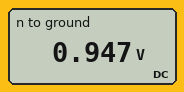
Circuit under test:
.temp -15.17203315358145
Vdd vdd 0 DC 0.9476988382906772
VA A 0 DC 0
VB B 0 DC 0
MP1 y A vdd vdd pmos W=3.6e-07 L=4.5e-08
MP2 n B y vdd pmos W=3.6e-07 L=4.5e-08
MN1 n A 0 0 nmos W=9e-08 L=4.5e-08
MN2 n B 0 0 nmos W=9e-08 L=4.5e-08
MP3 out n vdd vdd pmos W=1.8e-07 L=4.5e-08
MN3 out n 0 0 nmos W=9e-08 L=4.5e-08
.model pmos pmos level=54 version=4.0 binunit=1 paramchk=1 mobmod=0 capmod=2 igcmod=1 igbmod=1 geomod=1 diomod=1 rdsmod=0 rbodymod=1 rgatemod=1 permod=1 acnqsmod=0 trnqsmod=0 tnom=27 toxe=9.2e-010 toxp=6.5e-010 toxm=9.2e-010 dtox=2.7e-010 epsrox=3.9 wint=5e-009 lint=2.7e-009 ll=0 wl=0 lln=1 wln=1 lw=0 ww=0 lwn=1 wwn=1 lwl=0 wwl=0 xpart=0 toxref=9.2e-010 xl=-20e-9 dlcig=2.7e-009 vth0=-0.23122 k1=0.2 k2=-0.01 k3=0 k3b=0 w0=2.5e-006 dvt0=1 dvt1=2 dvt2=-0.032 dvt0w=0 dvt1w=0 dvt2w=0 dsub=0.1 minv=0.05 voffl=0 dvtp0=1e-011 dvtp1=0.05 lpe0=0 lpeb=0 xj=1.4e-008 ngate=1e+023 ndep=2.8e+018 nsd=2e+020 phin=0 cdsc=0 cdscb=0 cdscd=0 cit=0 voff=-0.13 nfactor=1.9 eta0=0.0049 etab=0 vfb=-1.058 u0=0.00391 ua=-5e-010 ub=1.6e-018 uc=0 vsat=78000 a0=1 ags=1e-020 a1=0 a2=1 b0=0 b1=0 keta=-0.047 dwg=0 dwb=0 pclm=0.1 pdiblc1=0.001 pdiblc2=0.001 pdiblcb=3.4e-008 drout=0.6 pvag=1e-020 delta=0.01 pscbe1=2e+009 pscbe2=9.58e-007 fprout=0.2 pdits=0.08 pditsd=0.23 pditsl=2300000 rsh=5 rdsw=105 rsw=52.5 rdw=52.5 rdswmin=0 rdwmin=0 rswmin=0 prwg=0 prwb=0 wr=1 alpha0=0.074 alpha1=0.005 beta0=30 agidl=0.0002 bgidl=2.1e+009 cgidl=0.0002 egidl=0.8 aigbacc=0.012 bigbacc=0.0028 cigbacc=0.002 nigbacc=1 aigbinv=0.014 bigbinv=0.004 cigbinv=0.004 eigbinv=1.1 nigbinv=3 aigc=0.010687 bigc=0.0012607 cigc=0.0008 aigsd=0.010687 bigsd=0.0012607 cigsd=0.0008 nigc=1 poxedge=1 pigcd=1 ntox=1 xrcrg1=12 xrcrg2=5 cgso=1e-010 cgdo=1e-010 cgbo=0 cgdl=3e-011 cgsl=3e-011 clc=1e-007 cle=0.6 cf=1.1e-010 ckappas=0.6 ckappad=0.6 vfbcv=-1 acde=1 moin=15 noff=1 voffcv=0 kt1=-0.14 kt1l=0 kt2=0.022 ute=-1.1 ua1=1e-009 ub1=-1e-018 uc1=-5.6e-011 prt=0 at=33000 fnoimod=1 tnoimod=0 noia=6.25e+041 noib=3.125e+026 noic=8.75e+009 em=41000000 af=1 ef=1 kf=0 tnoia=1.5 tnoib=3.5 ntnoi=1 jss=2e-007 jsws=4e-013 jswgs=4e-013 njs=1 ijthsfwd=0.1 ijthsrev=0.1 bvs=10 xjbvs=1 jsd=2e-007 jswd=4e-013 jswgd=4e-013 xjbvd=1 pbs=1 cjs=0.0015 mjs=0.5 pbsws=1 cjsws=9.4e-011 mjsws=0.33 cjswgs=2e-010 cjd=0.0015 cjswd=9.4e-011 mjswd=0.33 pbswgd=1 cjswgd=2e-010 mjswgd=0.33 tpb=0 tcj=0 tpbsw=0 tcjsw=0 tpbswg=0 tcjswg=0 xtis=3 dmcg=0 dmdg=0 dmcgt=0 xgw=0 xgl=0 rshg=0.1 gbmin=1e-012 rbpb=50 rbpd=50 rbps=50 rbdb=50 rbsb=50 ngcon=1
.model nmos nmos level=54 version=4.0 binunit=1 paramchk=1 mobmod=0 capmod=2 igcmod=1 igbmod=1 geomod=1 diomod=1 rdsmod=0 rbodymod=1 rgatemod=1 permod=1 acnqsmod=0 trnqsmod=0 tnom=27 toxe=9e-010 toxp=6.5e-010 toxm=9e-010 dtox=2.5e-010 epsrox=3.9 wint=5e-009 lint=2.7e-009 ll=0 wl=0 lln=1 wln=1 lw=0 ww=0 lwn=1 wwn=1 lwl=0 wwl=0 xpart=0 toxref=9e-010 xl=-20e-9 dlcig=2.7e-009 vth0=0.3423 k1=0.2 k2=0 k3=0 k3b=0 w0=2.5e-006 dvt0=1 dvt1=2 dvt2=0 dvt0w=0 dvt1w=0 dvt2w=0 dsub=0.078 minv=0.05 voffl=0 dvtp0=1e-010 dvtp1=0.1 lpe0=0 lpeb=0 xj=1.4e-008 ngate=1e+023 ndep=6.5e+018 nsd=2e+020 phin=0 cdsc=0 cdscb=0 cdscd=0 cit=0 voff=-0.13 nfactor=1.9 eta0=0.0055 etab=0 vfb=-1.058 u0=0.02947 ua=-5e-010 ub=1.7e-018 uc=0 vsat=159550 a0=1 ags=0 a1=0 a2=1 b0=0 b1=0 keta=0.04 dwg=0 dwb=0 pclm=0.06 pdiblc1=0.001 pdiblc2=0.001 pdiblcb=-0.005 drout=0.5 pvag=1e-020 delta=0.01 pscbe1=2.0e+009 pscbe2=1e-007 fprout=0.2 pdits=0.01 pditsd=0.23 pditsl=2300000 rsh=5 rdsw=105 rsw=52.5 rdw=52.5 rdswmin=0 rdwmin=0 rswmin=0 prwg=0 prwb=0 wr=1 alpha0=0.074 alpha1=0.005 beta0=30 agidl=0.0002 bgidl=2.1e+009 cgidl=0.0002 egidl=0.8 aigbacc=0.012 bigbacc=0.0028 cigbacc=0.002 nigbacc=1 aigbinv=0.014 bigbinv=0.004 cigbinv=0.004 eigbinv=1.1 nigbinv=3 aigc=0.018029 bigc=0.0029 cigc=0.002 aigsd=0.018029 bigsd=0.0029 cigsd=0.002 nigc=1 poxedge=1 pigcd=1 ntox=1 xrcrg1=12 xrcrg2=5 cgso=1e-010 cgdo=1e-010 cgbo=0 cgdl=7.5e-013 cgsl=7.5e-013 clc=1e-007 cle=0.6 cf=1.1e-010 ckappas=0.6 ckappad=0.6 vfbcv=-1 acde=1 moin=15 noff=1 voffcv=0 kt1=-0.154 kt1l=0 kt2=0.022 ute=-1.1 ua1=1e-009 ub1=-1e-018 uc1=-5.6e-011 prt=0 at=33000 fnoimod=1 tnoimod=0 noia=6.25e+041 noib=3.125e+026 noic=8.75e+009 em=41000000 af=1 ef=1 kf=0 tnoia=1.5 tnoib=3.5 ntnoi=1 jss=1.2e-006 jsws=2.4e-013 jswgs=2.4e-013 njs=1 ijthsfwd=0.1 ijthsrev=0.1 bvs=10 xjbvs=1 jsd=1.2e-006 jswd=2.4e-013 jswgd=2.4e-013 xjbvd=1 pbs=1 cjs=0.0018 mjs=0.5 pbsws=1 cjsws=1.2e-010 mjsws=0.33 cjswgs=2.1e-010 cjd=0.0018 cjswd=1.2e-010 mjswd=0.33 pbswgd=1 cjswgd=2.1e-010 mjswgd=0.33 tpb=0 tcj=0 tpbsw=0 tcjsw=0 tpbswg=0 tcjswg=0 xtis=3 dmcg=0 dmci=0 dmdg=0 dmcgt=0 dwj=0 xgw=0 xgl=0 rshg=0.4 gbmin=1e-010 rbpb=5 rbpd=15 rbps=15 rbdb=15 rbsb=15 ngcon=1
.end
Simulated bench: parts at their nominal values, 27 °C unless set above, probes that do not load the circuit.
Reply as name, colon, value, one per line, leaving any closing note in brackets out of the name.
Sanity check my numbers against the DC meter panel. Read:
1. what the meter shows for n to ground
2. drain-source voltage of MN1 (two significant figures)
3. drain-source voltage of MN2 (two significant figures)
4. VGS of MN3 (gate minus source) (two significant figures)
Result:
what the meter shows for n to ground: 0.947 V
drain-source voltage of MN1: 950 mV
drain-source voltage of MN2: 950 mV
VGS of MN3 (gate minus source): 950 mV
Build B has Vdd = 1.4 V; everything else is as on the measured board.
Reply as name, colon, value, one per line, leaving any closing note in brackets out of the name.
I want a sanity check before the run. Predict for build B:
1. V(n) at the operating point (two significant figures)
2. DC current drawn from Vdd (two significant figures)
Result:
V(n) at the operating point: 1.4 V
DC current drawn from Vdd: 2.9 µA
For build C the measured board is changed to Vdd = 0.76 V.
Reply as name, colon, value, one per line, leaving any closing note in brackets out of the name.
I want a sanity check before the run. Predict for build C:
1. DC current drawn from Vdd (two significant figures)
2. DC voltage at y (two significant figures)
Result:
DC current drawn from Vdd: 110 nA
DC voltage at y: 760 mV
